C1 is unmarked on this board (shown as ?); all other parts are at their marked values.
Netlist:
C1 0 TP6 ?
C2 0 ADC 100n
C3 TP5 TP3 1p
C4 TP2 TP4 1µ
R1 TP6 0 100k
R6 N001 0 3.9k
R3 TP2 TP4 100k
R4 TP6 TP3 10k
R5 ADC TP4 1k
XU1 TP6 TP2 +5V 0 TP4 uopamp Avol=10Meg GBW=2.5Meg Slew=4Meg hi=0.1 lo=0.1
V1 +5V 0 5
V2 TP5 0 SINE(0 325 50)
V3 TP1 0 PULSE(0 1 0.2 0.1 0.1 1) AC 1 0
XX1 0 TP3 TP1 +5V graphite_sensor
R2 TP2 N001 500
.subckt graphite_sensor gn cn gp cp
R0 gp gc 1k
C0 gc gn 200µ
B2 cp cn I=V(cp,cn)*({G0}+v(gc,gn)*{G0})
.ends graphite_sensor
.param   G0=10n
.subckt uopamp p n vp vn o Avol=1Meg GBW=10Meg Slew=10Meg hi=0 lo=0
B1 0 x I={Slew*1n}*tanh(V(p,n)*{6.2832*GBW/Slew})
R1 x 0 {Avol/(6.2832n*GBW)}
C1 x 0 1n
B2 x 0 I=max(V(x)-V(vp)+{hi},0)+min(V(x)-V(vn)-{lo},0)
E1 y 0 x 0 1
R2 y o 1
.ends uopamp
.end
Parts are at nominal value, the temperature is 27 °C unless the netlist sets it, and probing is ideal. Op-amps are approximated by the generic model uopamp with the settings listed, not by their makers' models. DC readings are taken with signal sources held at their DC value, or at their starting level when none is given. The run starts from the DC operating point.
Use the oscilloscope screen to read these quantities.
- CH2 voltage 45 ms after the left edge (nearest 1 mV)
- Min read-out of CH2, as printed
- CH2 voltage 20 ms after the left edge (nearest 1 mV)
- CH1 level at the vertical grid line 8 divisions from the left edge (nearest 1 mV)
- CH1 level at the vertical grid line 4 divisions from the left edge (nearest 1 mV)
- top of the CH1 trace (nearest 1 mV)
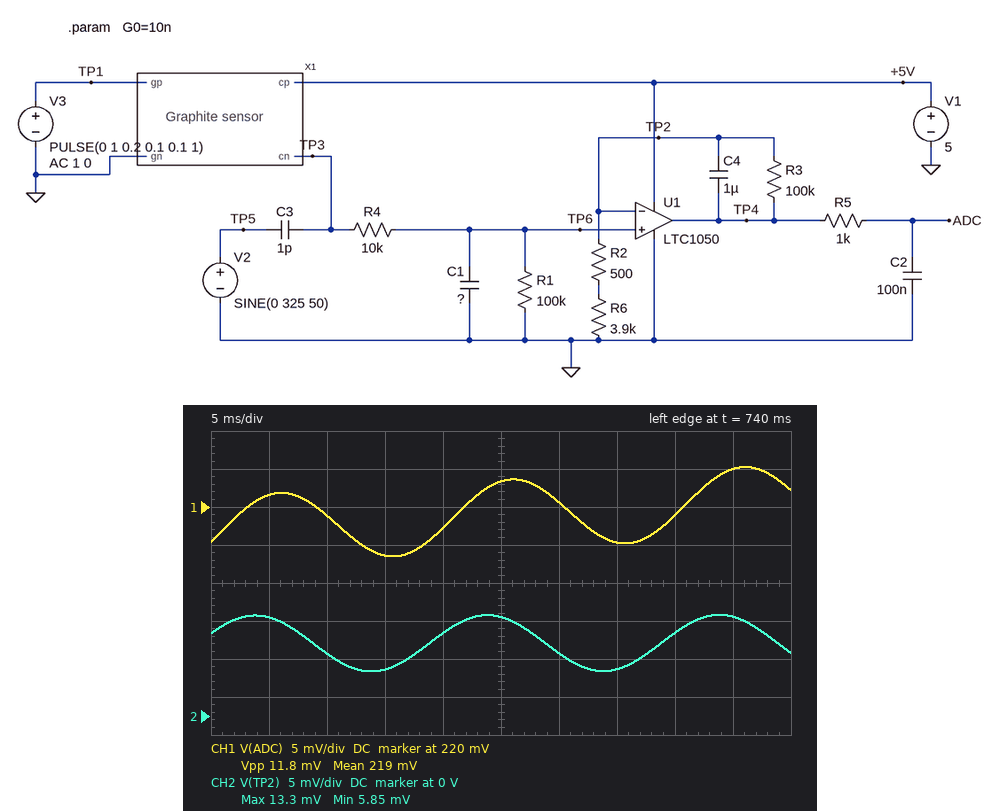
13 mV
5.85 mV
11 mV
219 mV
217 mV
225 mV
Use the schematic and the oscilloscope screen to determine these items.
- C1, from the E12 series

82 nF
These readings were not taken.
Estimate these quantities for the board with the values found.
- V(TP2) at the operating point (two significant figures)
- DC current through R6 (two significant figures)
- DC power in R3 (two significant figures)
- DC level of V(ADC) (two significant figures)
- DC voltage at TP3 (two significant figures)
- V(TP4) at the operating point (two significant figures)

5.0 mV
1.1 µA
130 nW
120 mV
5.5 mV
120 mV
